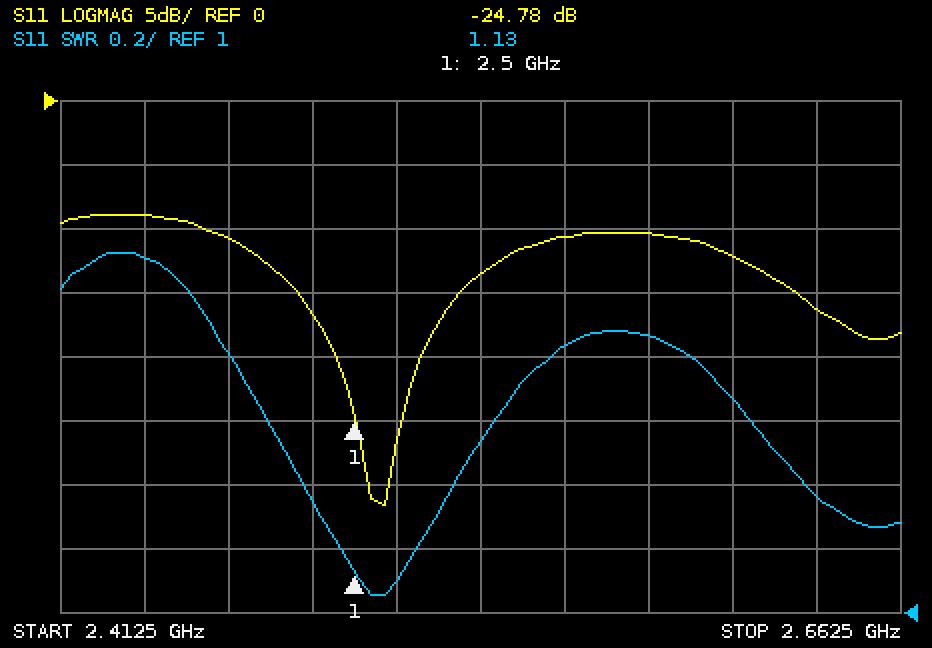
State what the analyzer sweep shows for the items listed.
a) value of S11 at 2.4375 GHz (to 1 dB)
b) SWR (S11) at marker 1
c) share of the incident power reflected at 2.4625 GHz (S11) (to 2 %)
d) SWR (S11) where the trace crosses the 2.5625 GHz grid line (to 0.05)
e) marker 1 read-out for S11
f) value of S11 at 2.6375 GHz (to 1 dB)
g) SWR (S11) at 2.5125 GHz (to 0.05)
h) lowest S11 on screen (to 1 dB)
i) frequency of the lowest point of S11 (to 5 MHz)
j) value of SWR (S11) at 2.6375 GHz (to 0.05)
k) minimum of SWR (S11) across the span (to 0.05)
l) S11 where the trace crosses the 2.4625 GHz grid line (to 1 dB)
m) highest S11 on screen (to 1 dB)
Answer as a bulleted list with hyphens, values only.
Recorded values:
- -9 dB
- 1.13
- 8 %
- 1.85
- -24.78 dB
- -16 dB
- 1.10
- -32 dB
- 2.510 GHz
- 1.35
- 1.05
- -11 dB
- -9 dB
